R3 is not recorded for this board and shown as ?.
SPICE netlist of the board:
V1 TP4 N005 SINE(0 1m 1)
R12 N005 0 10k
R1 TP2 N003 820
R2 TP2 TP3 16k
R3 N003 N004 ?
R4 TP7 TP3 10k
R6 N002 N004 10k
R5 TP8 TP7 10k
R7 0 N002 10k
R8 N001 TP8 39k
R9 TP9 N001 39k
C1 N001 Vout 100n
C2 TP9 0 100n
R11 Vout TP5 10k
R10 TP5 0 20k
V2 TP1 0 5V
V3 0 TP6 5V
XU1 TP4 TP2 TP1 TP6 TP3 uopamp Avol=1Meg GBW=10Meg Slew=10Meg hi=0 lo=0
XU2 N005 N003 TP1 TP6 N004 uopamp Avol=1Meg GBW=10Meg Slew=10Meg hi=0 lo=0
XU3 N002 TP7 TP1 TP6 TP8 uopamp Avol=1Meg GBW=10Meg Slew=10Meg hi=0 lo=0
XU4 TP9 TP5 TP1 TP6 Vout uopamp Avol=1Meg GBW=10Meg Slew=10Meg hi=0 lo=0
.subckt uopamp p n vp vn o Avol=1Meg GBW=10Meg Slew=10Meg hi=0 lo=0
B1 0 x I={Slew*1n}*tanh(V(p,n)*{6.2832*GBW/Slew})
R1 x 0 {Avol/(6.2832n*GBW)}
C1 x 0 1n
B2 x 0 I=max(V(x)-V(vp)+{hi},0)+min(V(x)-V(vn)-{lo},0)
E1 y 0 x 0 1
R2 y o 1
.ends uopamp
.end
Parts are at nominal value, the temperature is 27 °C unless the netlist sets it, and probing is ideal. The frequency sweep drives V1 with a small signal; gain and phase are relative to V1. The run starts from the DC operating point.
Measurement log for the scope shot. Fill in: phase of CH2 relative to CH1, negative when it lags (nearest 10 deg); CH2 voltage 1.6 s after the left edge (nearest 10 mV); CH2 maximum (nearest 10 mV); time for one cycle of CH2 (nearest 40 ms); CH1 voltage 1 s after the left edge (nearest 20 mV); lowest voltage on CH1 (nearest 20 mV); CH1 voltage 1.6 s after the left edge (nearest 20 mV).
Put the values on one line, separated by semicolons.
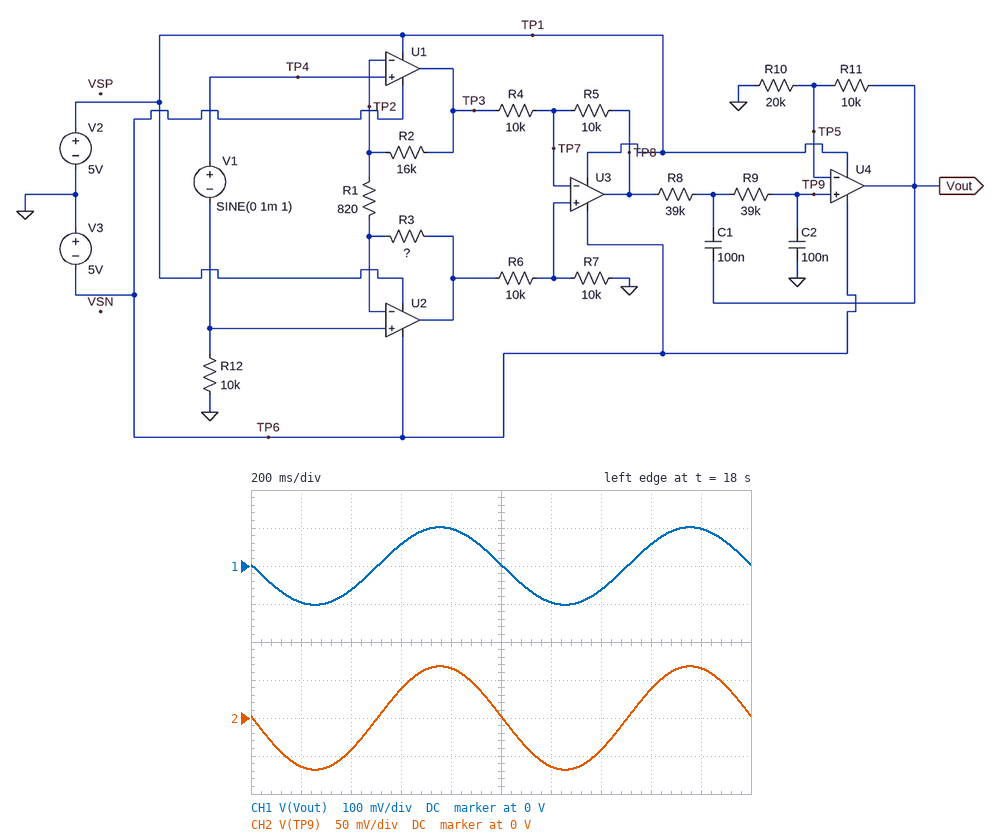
0 deg; 40 mV; 70 mV; 1.00 s; 0 V; -100 mV; 60 mV
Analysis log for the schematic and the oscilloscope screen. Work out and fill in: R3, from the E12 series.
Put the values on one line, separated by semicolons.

39 kΩ
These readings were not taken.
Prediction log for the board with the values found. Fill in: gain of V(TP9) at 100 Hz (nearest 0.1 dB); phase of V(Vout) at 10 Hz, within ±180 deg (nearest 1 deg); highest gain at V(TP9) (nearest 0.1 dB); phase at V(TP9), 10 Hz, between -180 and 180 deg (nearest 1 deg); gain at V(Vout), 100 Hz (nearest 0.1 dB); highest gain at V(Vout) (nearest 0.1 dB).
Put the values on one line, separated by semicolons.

20.8 dB; 159 deg; 36.7 dB; 159 deg; 24.3 dB; 40.2 dB
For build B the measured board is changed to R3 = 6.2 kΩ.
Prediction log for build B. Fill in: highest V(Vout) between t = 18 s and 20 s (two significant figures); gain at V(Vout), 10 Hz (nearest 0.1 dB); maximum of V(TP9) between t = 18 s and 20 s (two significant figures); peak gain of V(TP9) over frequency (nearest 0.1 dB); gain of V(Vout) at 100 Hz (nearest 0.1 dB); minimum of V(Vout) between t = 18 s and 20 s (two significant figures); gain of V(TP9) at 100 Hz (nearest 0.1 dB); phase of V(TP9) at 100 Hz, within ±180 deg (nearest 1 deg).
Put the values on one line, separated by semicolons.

42 mV; 32.4 dB; 28 mV; 29.0 dB; 16.6 dB; -42 mV; 13.1 dB; 36 deg
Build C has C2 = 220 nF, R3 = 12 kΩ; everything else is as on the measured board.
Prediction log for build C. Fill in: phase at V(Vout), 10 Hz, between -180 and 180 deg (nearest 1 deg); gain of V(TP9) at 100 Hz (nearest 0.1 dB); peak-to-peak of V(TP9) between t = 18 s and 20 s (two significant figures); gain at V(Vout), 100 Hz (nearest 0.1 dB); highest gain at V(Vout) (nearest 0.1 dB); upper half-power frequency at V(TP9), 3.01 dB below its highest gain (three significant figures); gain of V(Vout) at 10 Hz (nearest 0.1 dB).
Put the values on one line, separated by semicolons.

132 deg; 7.1 dB; 70 mV; 10.6 dB; 34.4 dB; 12.2 Hz; 32.2 dB
